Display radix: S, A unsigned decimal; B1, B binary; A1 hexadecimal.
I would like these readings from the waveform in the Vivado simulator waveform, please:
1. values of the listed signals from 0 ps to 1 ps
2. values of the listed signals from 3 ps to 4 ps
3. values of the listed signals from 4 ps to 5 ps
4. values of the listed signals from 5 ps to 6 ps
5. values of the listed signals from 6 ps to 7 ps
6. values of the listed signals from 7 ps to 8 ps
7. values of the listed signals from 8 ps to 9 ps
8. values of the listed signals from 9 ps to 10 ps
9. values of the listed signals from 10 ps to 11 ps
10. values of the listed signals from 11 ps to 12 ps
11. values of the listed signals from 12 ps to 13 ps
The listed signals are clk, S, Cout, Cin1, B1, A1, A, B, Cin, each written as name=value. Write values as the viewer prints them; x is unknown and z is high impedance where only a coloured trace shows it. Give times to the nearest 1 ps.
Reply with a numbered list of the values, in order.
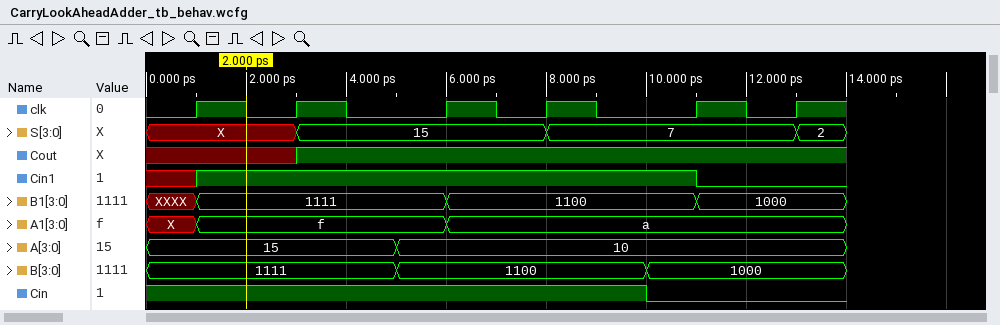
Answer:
1. clk=0, S=X, Cout=x, Cin1=x, B1=XXXX, A1=X, A=15, B=1111, Cin=1
2. clk=1, S=15, Cout=1, Cin1=1, B1=1111, A1=f, A=15, B=1111, Cin=1
3. clk=0, S=15, Cout=1, Cin1=1, B1=1111, A1=f, A=15, B=1111, Cin=1
4. clk=0, S=15, Cout=1, Cin1=1, B1=1111, A1=f, A=10, B=1100, Cin=1
5. clk=1, S=15, Cout=1, Cin1=1, B1=1100, A1=a, A=10, B=1100, Cin=1
6. clk=0, S=15, Cout=1, Cin1=1, B1=1100, A1=a, A=10, B=1100, Cin=1
7. clk=1, S=7, Cout=1, Cin1=1, B1=1100, A1=a, A=10, B=1100, Cin=1
8. clk=0, S=7, Cout=1, Cin1=1, B1=1100, A1=a, A=10, B=1100, Cin=1
9. clk=0, S=7, Cout=1, Cin1=1, B1=1100, A1=a, A=10, B=1000, Cin=0
10. clk=1, S=7, Cout=1, Cin1=0, B1=1000, A1=a, A=10, B=1000, Cin=0
11. clk=0, S=7, Cout=1, Cin1=0, B1=1000, A1=a, A=10, B=1000, Cin=0
